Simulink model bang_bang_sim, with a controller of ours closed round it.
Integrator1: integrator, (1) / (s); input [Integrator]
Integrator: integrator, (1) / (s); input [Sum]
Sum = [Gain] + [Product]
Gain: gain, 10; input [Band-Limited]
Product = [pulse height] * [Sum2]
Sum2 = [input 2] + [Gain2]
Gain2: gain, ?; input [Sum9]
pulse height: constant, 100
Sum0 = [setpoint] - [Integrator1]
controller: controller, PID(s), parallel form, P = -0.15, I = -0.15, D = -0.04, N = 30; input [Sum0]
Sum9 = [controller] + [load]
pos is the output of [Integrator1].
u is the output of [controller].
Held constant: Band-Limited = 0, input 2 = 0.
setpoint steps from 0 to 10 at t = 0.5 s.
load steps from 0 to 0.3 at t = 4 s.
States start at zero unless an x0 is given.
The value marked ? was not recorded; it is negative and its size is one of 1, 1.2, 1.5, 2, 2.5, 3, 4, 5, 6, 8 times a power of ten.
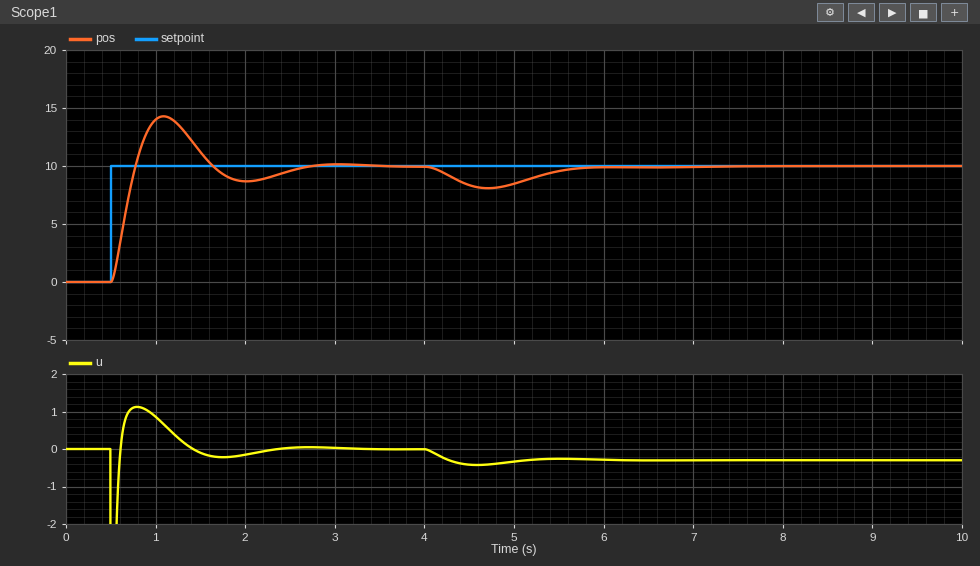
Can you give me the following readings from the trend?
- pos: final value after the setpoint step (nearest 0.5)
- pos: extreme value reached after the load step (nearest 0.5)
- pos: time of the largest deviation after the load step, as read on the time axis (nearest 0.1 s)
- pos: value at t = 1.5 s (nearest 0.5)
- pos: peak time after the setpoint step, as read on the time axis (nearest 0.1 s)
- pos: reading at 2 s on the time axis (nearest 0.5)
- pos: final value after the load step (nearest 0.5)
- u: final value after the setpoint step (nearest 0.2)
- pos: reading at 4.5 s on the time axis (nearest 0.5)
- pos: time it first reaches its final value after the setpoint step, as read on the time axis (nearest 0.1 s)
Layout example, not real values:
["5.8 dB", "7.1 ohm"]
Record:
["10.0", "8.0", "4.7 s", "11.0", "1.1 s", "8.5", "10.0", "0.0", "8.5", "0.8 s"]
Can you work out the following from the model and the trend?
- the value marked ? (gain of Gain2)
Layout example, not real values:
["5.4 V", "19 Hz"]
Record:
["-1"]
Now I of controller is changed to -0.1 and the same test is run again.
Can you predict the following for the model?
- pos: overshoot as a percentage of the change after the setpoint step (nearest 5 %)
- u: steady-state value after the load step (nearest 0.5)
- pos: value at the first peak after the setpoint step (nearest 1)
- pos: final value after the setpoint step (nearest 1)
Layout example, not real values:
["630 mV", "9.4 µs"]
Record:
["40 %", "-0.5", "14", "10"]
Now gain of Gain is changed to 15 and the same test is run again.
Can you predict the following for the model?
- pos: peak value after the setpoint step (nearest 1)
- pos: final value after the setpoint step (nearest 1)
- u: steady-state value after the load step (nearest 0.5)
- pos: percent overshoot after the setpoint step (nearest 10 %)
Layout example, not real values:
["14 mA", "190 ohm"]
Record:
["14", "10", "-0.5", "40 %"]
